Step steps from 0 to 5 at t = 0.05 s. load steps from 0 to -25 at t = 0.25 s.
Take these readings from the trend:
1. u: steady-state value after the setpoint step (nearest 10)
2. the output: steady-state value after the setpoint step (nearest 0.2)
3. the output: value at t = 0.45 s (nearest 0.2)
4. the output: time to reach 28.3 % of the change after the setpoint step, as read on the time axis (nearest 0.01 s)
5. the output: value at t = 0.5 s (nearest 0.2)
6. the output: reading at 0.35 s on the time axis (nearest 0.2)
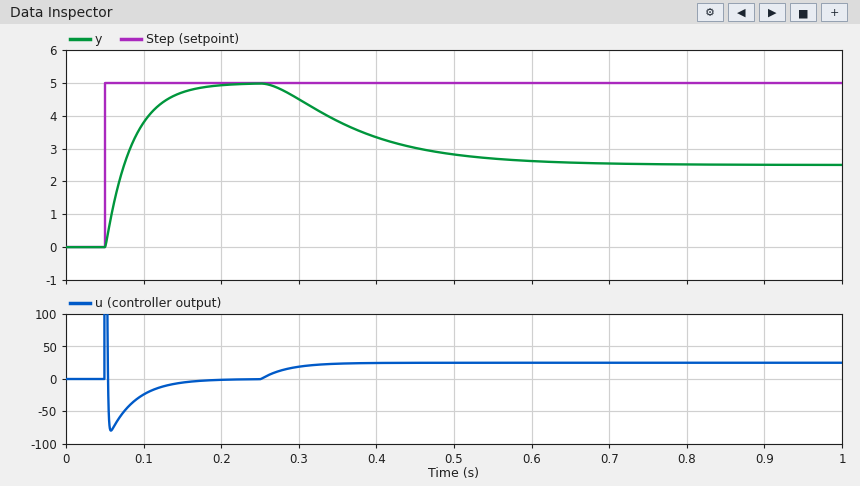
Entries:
0
5.0
3.0
0.06 s
2.8
3.8
